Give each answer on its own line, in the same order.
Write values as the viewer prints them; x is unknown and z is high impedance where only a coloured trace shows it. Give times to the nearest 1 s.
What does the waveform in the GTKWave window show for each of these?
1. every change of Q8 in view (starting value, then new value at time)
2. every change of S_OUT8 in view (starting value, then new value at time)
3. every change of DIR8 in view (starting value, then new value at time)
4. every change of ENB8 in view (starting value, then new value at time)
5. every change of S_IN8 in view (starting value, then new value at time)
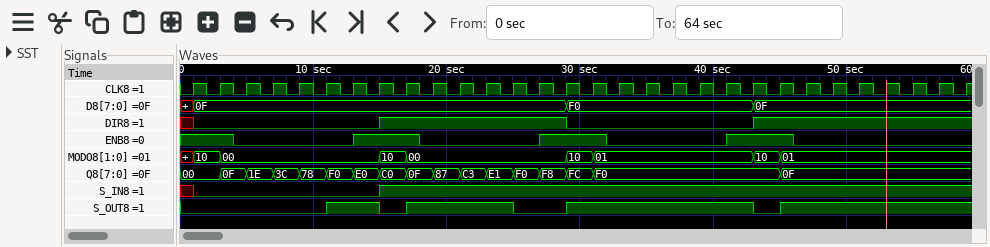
00, 0F at 3 s, 1E at 5 s, 3C at 7 s, 78 at 9 s, F0 at 11 s, E0 at 13 s, C0 at 15 s, 0F at 17 s, 87 at 19 s, C3 at 21 s, E1 at 23 s, F0 at 25 s, F8 at 27 s, FC at 29 s, F0 at 31 s, 0F at 45 s
0, 1 at 11 s, 0 at 15 s, 1 at 17 s, 0 at 25 s, 1 at 29 s, 0 at 43 s, 1 at 45 s
x, 0 at 1 s, 1 at 15 s, 0 at 29 s, 1 at 43 s
1, 0 at 4 s, 1 at 13 s, 0 at 18 s, 1 at 27 s, 0 at 32 s, 1 at 41 s, 0 at 46 s
x, 0 at 1 s, 1 at 15 s
